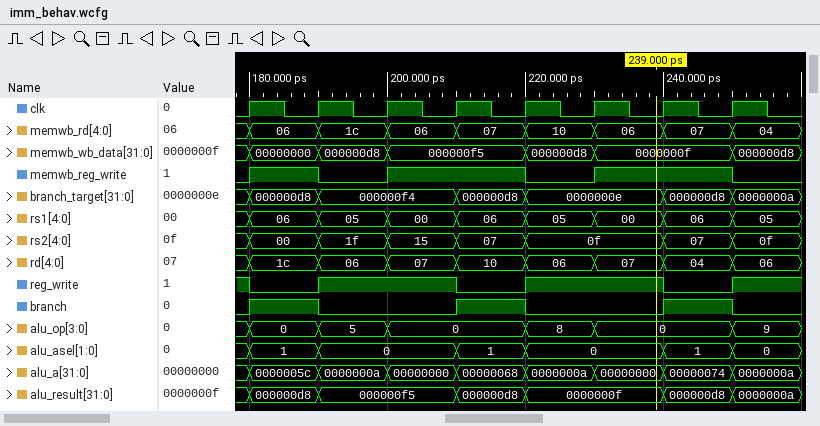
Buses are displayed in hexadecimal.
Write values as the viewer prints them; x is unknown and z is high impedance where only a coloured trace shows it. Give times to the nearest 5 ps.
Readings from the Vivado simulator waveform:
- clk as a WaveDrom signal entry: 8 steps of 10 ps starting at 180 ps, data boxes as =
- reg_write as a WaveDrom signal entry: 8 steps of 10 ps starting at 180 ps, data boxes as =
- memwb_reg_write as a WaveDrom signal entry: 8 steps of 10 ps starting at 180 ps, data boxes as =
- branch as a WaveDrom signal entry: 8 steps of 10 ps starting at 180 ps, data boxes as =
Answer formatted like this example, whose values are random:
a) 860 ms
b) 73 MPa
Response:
a) {name: 'clk', wave: 'p.......'}
b) {name: 'reg_write', wave: '01.01.01'}
c) {name: 'memwb_reg_write', wave: '101.01.0'}
d) {name: 'branch', wave: '10.10.10'}
